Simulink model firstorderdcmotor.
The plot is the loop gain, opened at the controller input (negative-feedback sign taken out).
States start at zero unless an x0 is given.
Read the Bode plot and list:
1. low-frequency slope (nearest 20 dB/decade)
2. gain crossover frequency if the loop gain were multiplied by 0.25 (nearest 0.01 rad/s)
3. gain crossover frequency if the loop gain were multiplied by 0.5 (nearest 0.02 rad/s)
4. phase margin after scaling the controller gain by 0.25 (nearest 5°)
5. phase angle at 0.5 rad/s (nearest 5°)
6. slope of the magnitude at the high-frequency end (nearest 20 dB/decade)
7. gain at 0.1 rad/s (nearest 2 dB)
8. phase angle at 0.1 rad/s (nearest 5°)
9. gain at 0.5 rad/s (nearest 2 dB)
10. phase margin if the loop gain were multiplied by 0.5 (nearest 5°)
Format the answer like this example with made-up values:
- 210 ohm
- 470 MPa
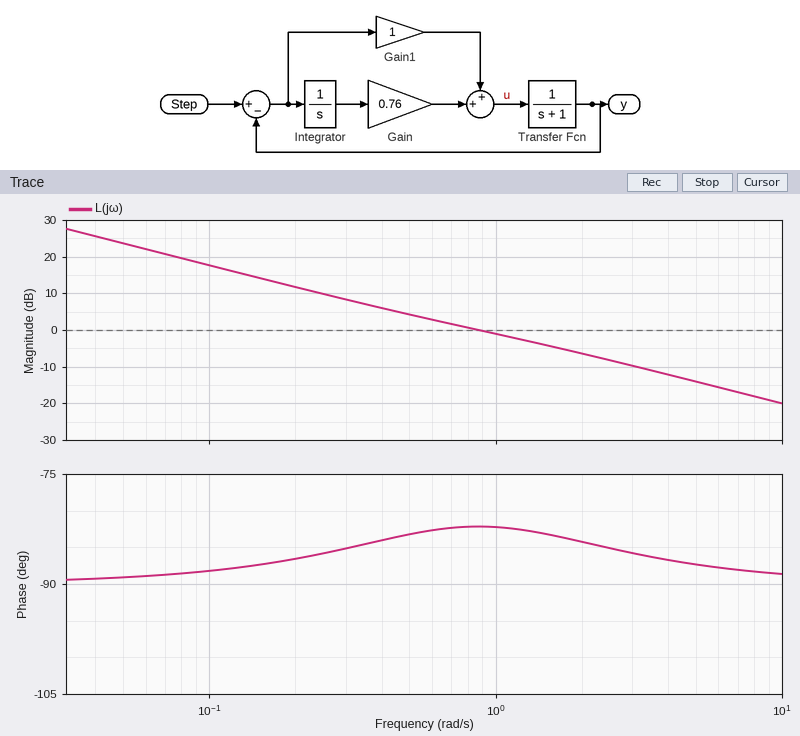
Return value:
- -20 dB/decade
- 0.19 rad/s
- 0.40 rad/s
- 95°
- -85°
- -20 dB/decade
- 18 dB
- -90°
- 4 dB
- 95°
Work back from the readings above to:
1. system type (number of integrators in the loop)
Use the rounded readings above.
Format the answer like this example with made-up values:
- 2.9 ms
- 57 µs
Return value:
- 1
